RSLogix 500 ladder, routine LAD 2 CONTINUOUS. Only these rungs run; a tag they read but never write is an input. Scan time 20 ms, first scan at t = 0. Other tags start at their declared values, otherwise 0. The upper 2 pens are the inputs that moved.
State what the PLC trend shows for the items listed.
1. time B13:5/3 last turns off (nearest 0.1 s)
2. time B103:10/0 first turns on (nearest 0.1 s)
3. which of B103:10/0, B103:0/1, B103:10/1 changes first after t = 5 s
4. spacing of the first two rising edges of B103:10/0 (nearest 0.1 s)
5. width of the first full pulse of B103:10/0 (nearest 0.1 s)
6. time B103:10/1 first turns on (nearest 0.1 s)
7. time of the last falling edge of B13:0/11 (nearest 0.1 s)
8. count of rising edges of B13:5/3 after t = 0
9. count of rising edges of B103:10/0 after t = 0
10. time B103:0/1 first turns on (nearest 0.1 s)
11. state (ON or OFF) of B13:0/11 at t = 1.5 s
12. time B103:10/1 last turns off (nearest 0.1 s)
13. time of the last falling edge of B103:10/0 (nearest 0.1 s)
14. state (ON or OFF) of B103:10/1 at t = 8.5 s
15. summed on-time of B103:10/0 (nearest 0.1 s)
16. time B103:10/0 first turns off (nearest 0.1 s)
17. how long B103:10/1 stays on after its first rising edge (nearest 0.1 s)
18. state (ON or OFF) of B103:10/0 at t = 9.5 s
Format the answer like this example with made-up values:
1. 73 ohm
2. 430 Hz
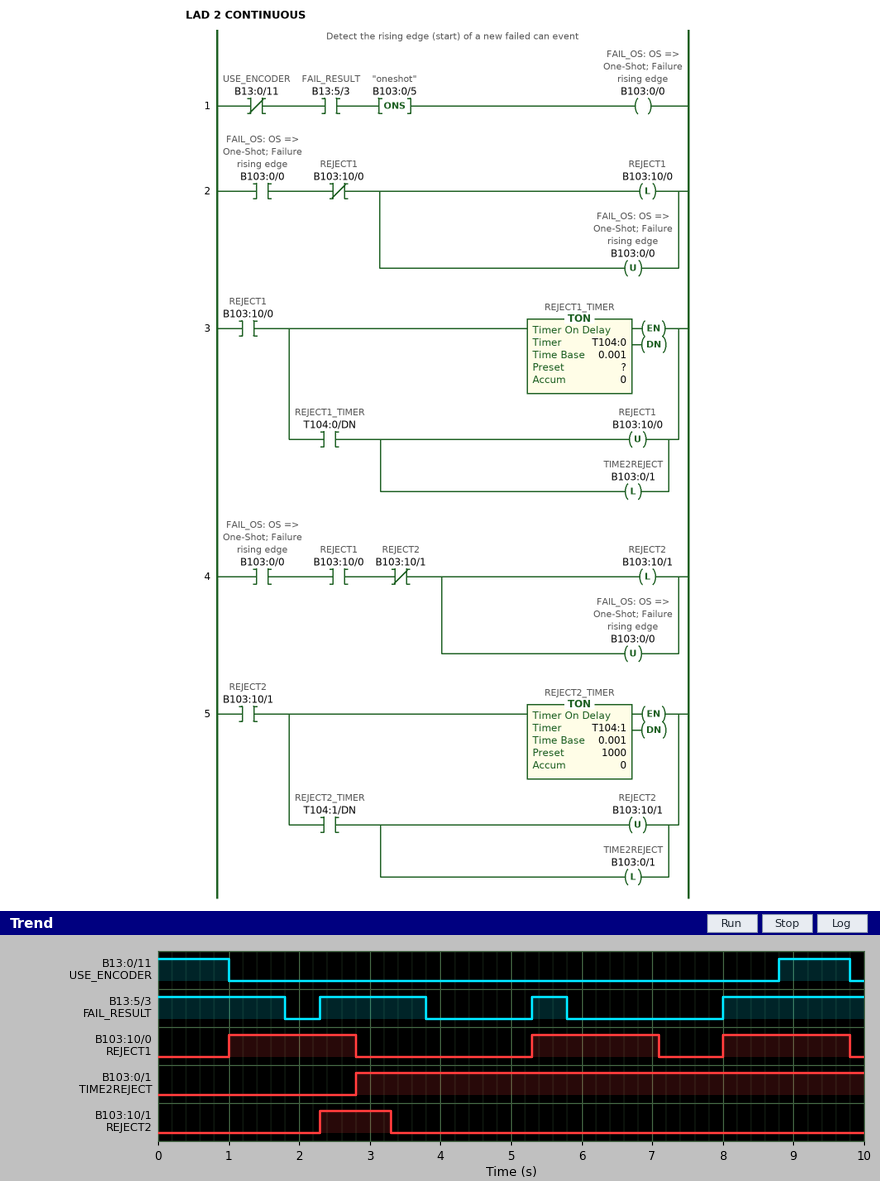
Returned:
1. 5.8 s
2. 1.0 s
3. B103:10/0
4. 4.3 s
5. 1.8 s
6. 2.3 s
7. 9.8 s
8. 3
9. 3
10. 2.8 s
11. OFF
12. 3.3 s
13. 9.8 s
14. OFF
15. 5.4 s
16. 2.8 s
17. 1.0 s
18. ON
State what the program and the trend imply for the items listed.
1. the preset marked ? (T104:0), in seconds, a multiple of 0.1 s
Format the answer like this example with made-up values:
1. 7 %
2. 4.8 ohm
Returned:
1. 1.8 s
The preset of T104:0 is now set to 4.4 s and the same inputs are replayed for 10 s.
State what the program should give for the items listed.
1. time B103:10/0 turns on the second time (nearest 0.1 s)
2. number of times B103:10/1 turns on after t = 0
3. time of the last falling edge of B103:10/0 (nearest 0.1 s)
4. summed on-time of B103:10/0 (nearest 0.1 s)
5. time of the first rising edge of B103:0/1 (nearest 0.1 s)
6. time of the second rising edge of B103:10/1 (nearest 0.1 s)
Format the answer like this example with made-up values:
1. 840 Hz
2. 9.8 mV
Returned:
1. 8.0 s
2. 3
3. 5.4 s
4. 6.4 s
5. 3.3 s
6. 5.3 s
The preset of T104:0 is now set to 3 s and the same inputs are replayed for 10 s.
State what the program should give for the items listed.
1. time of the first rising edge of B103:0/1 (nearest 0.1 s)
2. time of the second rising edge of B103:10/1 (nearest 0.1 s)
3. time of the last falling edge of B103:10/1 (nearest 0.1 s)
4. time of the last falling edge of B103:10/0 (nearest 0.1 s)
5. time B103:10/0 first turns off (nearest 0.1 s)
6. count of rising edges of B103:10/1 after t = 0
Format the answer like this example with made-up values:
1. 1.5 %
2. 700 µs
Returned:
1. 3.3 s
2. 8.0 s
3. 9.0 s
4. 8.3 s
5. 4.0 s
6. 2
